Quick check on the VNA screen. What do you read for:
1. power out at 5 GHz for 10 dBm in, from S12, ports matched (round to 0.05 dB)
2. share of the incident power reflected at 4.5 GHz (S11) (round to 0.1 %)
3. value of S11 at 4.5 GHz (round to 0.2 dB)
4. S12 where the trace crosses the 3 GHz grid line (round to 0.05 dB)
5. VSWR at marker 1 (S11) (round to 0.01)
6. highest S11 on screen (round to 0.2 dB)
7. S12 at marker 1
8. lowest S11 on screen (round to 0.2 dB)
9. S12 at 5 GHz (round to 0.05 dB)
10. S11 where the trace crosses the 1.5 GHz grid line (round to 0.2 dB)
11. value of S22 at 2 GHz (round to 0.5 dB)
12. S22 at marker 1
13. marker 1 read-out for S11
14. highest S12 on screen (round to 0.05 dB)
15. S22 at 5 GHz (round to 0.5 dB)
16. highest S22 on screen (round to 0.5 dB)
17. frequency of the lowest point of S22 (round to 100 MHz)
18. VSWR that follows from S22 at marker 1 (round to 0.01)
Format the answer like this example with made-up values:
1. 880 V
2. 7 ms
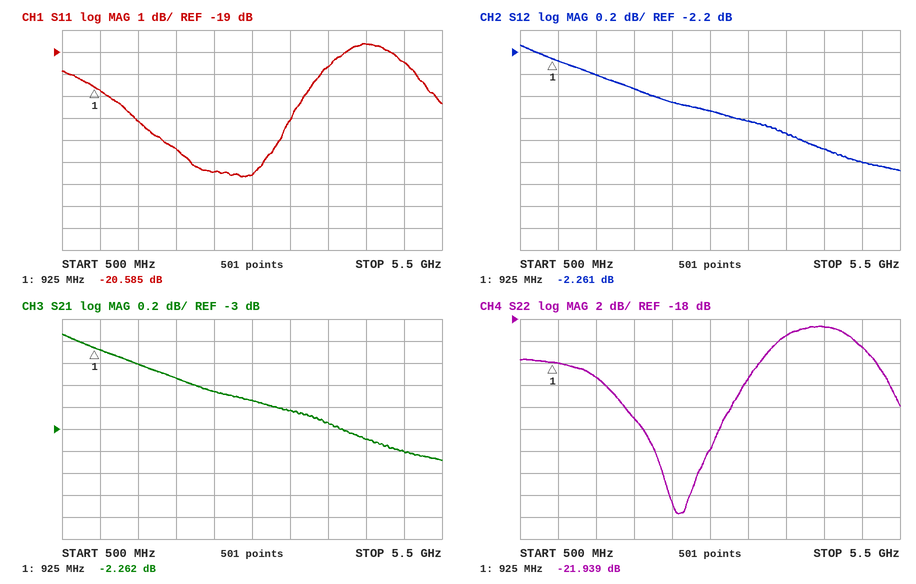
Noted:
1. 6.80 dBm
2. 1.4 %
3. -18.6 dB
4. -2.75 dB
5. 1.21
6. -18.6 dB
7. -2.261 dB
8. -24.6 dB
9. -3.20 dB
10. -22.2 dB
11. -27.0 dB
12. -21.939 dB
13. -20.585 dB
14. -2.15 dB
15. -20.5 dB
16. -18.5 dB
17. 2.6 GHz
18. 1.17
